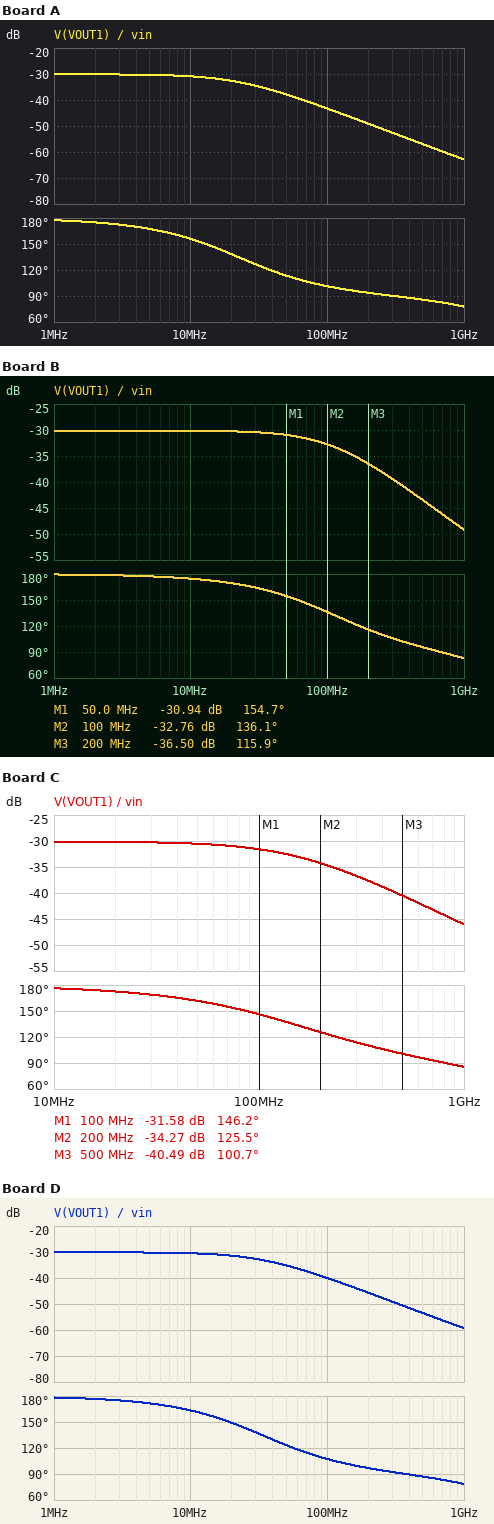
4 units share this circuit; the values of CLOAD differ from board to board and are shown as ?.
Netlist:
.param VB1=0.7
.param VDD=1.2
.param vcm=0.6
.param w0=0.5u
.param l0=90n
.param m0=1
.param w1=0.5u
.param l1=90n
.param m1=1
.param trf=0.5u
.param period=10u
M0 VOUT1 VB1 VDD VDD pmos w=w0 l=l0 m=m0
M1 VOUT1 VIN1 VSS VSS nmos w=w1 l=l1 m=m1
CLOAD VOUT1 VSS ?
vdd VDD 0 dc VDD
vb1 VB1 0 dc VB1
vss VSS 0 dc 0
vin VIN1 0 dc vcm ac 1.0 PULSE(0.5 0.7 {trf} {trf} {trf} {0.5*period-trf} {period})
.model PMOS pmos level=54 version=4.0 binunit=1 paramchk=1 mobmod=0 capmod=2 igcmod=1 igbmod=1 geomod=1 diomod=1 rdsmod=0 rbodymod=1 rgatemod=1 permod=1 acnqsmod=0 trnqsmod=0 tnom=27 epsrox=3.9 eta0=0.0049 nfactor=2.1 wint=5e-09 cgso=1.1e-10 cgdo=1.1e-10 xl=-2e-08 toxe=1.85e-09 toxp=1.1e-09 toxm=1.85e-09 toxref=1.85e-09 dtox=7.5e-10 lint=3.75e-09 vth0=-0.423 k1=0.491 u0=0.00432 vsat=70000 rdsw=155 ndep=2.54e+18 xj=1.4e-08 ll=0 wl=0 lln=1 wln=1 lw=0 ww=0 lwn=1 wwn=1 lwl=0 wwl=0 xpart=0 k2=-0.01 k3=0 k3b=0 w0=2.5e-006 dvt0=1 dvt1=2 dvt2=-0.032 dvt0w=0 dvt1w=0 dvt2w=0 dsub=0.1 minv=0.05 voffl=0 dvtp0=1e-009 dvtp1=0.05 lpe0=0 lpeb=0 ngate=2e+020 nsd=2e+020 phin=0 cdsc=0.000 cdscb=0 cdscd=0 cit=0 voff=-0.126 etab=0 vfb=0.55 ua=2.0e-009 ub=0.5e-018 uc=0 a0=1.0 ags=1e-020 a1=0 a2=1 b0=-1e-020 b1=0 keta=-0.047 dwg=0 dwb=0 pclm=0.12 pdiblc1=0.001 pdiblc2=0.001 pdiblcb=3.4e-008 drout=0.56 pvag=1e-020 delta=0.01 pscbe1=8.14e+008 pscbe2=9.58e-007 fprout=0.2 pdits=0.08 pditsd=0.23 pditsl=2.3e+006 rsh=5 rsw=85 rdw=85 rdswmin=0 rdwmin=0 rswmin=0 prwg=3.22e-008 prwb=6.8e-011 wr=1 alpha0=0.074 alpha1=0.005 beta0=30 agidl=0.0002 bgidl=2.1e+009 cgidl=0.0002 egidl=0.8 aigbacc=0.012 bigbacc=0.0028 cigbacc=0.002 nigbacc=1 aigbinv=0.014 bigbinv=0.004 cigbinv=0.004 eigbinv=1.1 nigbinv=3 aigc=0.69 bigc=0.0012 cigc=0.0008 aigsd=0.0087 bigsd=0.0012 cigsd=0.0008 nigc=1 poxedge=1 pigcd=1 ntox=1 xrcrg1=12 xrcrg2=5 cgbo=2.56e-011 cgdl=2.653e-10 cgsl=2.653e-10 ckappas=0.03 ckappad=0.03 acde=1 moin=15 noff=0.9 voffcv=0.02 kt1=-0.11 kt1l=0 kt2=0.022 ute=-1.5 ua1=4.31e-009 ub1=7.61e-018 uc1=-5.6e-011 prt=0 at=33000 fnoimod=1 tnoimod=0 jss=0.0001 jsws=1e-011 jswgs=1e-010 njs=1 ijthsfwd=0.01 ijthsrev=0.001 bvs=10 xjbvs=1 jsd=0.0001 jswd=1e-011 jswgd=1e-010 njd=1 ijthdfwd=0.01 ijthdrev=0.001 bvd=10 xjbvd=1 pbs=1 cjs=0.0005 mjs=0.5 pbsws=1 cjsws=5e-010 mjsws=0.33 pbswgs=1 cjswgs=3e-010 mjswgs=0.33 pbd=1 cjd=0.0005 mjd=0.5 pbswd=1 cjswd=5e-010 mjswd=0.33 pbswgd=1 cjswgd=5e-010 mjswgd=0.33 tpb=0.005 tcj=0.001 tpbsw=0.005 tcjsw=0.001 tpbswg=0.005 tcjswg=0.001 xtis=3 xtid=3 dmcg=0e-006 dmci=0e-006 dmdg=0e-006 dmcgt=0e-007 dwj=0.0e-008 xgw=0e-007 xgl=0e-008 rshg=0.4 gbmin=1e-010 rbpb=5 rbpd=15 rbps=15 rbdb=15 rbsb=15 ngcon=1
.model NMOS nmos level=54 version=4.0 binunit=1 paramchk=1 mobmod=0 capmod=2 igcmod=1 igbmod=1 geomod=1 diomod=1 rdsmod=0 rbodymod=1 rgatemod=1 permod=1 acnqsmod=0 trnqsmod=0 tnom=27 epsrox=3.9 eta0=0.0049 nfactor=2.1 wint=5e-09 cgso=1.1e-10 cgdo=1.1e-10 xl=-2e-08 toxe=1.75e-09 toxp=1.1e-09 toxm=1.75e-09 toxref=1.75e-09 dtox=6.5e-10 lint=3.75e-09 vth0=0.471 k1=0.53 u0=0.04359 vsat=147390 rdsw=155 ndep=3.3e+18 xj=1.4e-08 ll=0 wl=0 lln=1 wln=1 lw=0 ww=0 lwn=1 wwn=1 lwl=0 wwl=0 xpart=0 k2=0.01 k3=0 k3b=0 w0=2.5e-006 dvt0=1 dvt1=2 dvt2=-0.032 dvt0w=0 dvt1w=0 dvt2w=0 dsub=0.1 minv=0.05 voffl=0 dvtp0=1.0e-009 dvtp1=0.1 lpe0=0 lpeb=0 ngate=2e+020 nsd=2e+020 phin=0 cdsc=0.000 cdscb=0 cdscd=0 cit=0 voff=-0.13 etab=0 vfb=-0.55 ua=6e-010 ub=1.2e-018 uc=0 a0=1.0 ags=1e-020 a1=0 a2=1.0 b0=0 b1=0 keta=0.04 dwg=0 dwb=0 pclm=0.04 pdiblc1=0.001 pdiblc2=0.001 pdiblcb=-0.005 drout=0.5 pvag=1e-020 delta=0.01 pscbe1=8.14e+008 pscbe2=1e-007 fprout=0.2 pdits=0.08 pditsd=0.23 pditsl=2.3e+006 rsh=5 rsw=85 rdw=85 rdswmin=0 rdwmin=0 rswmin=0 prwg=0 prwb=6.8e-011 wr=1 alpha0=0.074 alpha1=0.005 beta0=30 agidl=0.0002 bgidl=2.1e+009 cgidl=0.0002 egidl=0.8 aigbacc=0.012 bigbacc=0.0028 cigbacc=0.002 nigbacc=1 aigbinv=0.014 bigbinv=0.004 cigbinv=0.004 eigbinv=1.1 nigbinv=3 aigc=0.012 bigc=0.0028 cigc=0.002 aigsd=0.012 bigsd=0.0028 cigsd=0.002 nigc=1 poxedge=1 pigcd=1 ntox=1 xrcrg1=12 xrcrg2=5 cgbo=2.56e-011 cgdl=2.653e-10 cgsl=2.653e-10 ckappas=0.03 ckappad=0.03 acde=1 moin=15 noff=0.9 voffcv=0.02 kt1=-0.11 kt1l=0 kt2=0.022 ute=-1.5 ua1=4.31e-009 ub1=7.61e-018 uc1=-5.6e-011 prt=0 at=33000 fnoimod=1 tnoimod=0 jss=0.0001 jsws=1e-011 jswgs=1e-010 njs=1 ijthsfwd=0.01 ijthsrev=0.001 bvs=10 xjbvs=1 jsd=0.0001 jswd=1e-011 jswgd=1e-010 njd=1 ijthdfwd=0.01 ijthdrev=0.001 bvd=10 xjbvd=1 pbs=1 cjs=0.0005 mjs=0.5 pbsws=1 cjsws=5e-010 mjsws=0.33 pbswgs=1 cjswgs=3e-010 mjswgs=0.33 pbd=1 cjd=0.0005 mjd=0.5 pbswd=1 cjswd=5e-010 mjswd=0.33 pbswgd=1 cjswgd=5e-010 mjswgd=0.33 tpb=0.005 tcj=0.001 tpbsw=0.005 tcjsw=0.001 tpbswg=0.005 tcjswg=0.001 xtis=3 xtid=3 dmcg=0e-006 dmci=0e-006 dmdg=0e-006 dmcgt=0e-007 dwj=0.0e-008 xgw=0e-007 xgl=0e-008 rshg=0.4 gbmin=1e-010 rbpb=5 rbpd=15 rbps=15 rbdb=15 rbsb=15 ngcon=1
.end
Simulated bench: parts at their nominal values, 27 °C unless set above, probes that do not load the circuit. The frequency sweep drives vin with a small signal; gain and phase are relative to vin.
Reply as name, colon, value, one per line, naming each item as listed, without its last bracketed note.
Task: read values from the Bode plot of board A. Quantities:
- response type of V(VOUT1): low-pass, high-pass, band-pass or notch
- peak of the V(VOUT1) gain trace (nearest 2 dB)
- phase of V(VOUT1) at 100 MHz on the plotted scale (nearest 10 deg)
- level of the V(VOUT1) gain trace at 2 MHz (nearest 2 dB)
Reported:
response type of V(VOUT1): low-pass, high-pass, band-pass or notch: low-pass
peak of the V(VOUT1) gain trace: -30 dB
phase of V(VOUT1) at 100 MHz on the plotted scale: 100 deg
level of the V(VOUT1) gain trace at 2 MHz: -30 dB
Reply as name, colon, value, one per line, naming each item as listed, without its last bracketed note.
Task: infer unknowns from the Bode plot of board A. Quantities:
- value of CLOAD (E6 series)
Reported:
value of CLOAD: 3.3 pF
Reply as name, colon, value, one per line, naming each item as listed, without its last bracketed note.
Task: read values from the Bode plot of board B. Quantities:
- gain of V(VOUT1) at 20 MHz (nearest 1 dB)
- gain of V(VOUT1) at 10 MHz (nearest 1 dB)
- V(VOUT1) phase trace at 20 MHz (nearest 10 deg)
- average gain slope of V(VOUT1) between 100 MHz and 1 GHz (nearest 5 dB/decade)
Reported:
gain of V(VOUT1) at 20 MHz: -30 dB
gain of V(VOUT1) at 10 MHz: -30 dB
V(VOUT1) phase trace at 20 MHz: 170 deg
average gain slope of V(VOUT1) between 100 MHz and 1 GHz: -15 dB/decade
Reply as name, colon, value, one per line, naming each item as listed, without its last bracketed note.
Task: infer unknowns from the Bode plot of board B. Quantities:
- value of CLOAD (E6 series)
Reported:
value of CLOAD: 680 fF
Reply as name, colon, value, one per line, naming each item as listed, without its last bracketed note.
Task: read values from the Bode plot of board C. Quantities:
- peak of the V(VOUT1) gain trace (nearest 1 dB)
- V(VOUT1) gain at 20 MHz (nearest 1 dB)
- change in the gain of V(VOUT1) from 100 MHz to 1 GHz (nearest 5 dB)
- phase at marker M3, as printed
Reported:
peak of the V(VOUT1) gain trace: -30 dB
V(VOUT1) gain at 20 MHz: -30 dB
change in the gain of V(VOUT1) from 100 MHz to 1 GHz: -15 dB
phase at marker M3, as printed: 100.7 deg
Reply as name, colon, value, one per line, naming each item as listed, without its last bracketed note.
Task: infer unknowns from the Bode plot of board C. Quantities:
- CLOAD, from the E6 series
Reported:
CLOAD, from the E6 series: 470 fF
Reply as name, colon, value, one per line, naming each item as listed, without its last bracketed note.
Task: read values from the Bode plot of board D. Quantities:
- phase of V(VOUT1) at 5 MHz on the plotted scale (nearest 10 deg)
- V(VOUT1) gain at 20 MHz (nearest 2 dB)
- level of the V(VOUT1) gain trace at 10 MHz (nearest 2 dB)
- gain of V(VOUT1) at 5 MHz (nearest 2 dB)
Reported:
phase of V(VOUT1) at 5 MHz on the plotted scale: 170 deg
V(VOUT1) gain at 20 MHz: -32 dB
level of the V(VOUT1) gain trace at 10 MHz: -30 dB
gain of V(VOUT1) at 5 MHz: -30 dB
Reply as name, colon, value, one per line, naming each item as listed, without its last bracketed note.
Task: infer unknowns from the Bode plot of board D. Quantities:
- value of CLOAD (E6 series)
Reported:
value of CLOAD: 2.2 pF
